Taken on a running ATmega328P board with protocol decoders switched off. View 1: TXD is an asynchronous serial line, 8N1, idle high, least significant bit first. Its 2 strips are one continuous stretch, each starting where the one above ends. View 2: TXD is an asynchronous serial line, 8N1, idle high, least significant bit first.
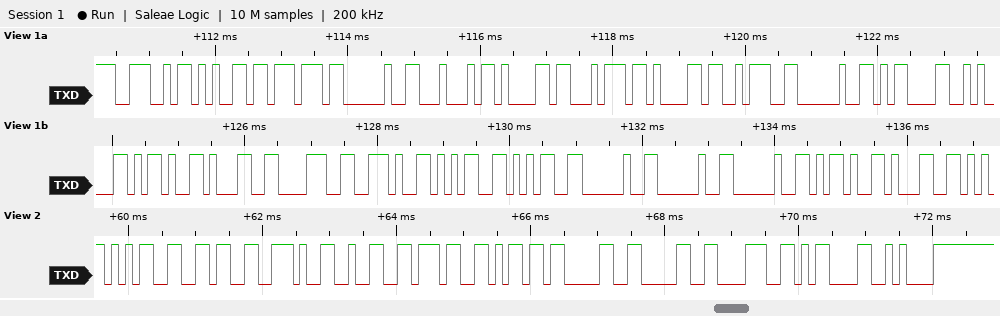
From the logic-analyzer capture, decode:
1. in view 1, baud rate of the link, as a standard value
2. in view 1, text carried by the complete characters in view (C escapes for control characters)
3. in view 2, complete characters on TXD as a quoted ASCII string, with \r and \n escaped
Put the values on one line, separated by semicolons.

9600 baud; "New Data: \r\n-18.55   -1"; "56.27m008\r\n"
